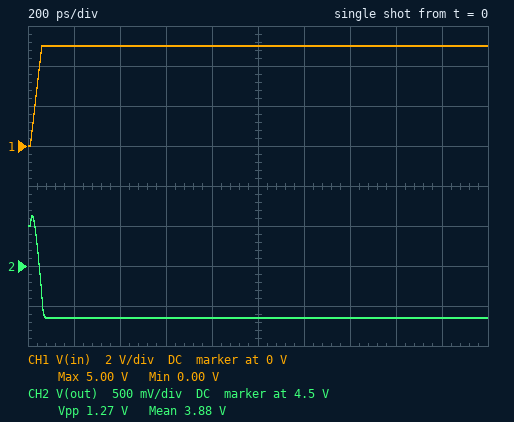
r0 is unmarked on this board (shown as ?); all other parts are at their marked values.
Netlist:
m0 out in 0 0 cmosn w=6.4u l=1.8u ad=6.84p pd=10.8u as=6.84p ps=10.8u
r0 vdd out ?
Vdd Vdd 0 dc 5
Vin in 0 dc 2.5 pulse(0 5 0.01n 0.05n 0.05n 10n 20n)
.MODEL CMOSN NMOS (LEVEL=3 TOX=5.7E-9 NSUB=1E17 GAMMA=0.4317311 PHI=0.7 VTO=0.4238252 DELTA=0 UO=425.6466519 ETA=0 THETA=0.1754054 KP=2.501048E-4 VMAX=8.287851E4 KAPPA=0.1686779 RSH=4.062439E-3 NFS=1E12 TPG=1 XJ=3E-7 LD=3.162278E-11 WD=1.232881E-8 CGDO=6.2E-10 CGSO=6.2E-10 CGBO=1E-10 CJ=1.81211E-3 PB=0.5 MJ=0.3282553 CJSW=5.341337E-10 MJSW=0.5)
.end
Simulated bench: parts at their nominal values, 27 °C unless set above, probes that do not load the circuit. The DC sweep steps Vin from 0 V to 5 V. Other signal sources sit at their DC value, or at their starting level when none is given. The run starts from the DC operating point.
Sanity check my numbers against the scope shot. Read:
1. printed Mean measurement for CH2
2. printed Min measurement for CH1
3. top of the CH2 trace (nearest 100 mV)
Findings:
3.88 V
0.00 V
5.1 V
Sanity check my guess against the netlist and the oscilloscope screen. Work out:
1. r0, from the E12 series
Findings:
390 Ω
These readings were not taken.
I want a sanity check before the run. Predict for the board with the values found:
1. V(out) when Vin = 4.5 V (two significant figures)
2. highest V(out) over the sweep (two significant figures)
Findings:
4.0 V
5.0 V
